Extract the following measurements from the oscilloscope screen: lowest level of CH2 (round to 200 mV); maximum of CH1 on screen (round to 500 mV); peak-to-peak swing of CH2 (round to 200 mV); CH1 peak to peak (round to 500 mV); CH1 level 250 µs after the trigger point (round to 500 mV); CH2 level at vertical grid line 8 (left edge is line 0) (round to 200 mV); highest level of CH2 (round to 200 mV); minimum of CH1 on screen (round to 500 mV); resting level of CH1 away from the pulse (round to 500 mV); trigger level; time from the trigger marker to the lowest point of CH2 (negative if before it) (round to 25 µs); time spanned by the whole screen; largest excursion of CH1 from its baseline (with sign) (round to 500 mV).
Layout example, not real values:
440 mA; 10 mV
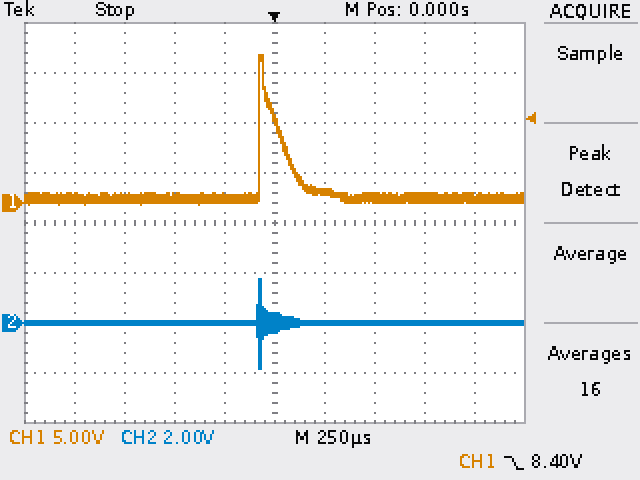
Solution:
-1.8 V; 15.0 V; 3.6 V; 15.0 V; 1.0 V; 0.0 V; 1.8 V; 0.0 V; 500 mV; 8.40 V; -75 µs; 2.5 ms; +14.5 V
